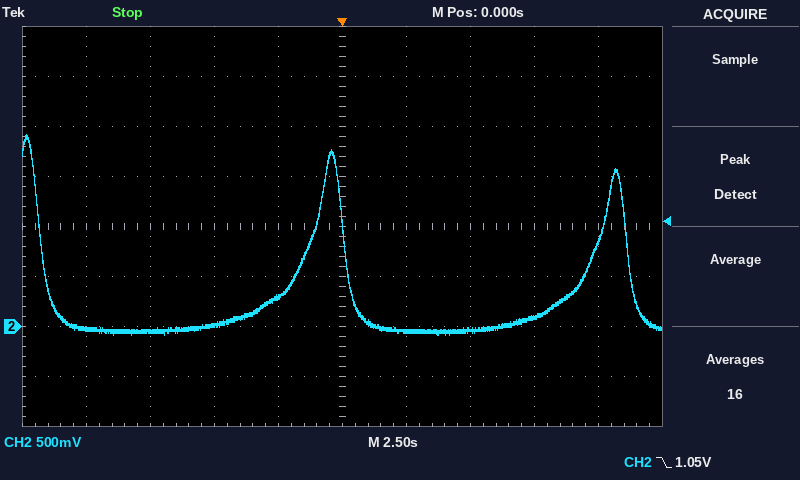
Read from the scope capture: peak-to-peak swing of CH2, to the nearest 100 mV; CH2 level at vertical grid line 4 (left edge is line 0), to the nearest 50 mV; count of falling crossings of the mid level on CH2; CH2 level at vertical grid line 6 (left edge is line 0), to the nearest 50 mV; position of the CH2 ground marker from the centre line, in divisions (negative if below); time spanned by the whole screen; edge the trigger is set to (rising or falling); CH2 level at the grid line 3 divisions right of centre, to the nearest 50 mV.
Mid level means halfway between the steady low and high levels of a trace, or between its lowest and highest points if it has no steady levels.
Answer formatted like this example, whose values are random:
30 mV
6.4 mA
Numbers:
2.00 V
300 mV
3
-50 mV
-2.0 div
25 s
falling
100 mV
